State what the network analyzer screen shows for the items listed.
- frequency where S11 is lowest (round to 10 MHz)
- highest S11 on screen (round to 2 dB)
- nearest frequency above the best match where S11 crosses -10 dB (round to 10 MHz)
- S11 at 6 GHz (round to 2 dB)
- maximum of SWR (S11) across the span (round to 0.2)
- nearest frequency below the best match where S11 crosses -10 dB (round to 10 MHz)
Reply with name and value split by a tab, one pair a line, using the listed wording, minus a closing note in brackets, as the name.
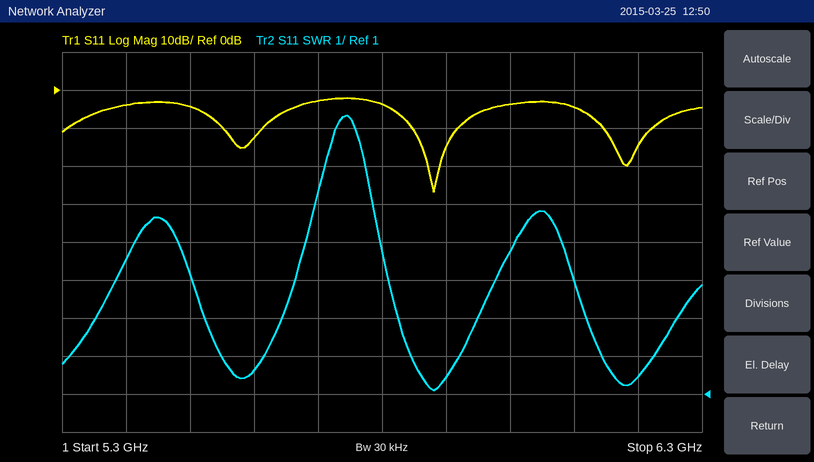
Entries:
frequency where S11 is lowest	5.88 GHz
highest S11 on screen	-2 dB
nearest frequency above the best match where S11 crosses -10 dB	5.92 GHz
S11 at 6 GHz	-4 dB
maximum of SWR (S11) across the span	8.4
nearest frequency below the best match where S11 crosses -10 dB	5.85 GHz
